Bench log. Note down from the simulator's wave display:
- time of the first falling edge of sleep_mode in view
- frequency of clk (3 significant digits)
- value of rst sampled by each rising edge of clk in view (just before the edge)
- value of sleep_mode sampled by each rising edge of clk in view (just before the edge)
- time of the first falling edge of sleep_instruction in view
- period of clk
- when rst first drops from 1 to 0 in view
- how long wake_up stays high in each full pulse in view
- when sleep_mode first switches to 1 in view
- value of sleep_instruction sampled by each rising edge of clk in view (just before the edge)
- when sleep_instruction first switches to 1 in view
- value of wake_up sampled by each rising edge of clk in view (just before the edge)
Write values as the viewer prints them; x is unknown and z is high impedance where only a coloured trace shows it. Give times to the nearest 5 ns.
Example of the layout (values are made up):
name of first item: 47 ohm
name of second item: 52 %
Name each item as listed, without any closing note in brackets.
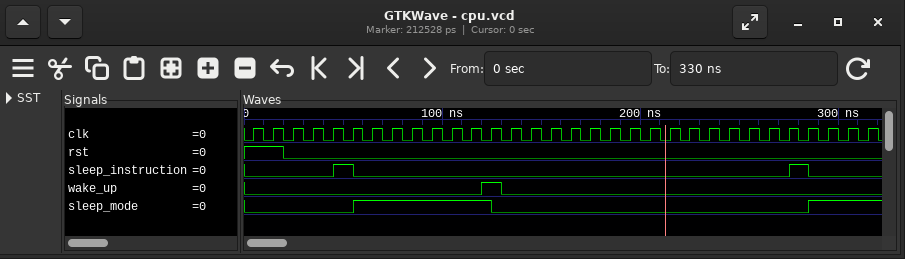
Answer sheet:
time of the first falling edge of sleep_mode in view: 125 ns
frequency of clk: 100 MHz
value of rst sampled by each rising edge of clk in view: 1 1 0 0 0 0 0 0 0 0 0 0 0 0 0 0 0 0 0 0 0 0 0 0 0 0 0 0 0 0 0 0
value of sleep_mode sampled by each rising edge of clk in view: 0 0 0 0 0 0 1 1 1 1 1 1 1 0 0 0 0 0 0 0 0 0 0 0 0 0 0 0 0 1 1 1
time of the first falling edge of sleep_instruction in view: 55 ns
period of clk: 10 ns
when rst first drops from 1 to 0 in view: 20 ns
how long wake_up stays high in each full pulse in view: 10 ns
when sleep_mode first switches to 1 in view: 55 ns
value of sleep_instruction sampled by each rising edge of clk in view: 0 0 0 0 0 1 0 0 0 0 0 0 0 0 0 0 0 0 0 0 0 0 0 0 0 0 0 0 1 0 0 0
when sleep_instruction first switches to 1 in view: 45 ns
value of wake_up sampled by each rising edge of clk in view: 0 0 0 0 0 0 0 0 0 0 0 0 1 0 0 0 0 0 0 0 0 0 0 0 0 0 0 0 0 0 0 0
